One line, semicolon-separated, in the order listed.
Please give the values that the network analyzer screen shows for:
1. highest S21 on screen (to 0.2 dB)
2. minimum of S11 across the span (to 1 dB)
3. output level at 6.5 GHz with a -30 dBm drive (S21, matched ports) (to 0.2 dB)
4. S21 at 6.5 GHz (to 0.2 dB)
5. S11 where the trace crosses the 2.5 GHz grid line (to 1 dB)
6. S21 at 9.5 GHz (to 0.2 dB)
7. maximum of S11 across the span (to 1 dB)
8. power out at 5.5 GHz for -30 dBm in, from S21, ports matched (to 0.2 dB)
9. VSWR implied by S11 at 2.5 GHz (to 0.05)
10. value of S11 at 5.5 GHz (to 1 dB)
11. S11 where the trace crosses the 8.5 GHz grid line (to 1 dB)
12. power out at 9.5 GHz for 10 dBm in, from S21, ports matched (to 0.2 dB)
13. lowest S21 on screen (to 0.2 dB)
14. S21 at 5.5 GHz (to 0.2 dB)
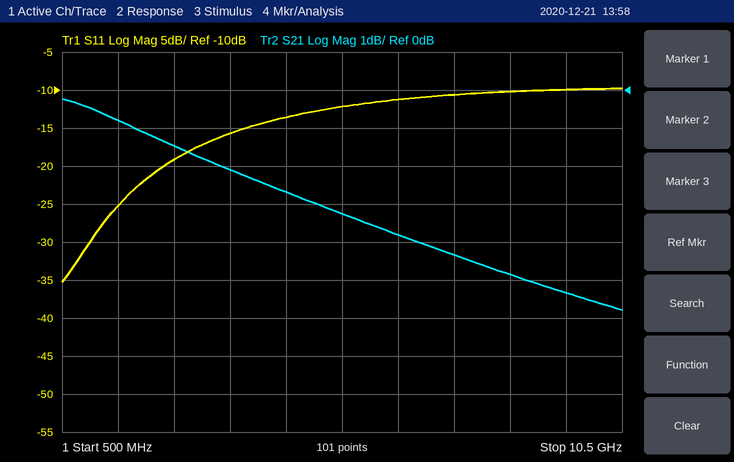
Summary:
-0.2 dB; -35 dB; -33.8 dBm; -3.8 dB; -19 dB; -5.4 dB; -10 dB; -33.2 dBm; 1.25; -12 dB; -10 dB; 4.6 dBm; -5.8 dB; -3.2 dB
